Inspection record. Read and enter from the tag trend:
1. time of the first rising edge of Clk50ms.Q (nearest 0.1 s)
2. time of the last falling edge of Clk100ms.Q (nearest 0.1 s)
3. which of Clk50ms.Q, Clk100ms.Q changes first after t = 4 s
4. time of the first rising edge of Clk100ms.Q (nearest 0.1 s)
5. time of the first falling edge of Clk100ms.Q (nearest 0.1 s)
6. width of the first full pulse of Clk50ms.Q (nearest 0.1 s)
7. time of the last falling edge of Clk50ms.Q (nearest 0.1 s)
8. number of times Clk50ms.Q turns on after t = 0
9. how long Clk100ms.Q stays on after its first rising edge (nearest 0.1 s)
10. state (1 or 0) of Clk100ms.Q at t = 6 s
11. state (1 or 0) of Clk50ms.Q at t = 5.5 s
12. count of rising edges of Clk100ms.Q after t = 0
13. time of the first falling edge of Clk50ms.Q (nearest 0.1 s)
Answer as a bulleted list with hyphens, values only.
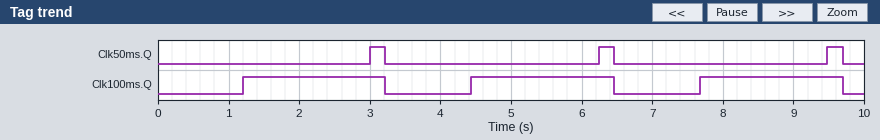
- 3.0 s
- 9.7 s
- Clk100ms.Q
- 1.2 s
- 3.2 s
- 0.2 s
- 9.7 s
- 3
- 2.0 s
- 1
- 0
- 3
- 3.2 s
